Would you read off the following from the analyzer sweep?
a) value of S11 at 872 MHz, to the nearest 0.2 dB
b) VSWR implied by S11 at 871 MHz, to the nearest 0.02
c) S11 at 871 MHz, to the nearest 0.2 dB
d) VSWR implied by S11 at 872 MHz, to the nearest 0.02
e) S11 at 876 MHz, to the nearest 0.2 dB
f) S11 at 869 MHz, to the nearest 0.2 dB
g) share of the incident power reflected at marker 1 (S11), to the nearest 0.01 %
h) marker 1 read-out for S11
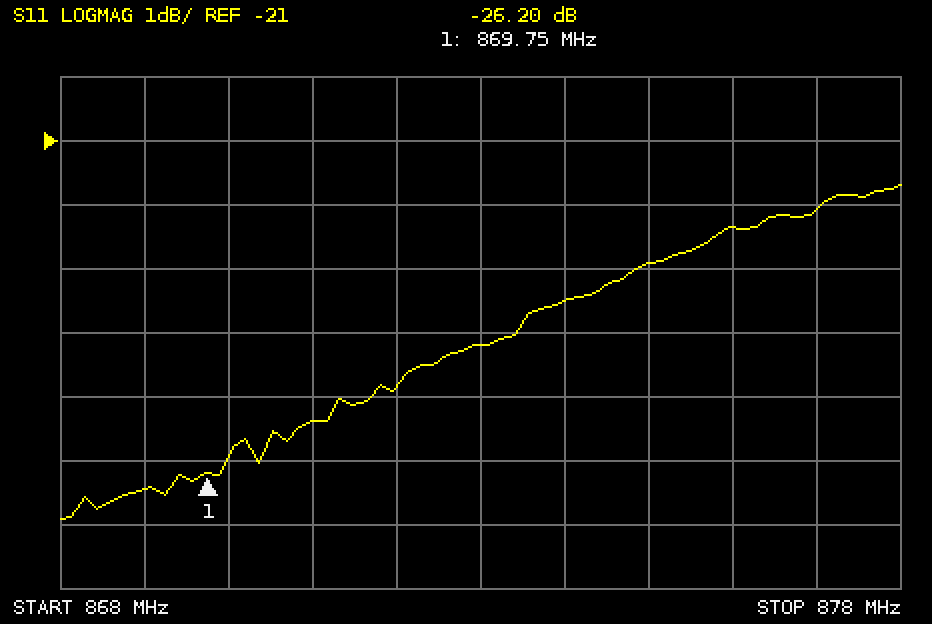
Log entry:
-24.8 dB
1.12
-25.4 dB
1.12
-22.4 dB
-26.4 dB
0.24 %
-26.20 dB
